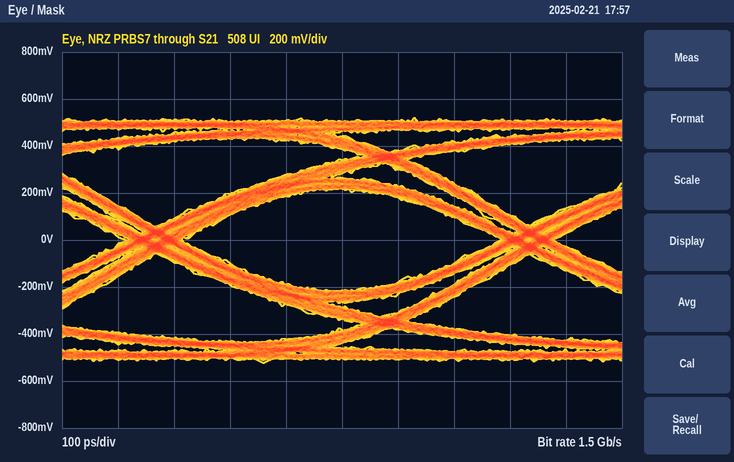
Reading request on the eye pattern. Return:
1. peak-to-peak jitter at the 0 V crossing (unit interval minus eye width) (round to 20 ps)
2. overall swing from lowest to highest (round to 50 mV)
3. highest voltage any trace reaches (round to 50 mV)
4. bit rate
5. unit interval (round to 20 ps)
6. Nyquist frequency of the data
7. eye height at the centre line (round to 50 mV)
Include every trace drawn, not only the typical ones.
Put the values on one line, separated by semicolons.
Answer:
100 ps; 1.05 V; 500 mV; 1.5 Gb/s; 660 ps; 750 MHz; 450 mV
